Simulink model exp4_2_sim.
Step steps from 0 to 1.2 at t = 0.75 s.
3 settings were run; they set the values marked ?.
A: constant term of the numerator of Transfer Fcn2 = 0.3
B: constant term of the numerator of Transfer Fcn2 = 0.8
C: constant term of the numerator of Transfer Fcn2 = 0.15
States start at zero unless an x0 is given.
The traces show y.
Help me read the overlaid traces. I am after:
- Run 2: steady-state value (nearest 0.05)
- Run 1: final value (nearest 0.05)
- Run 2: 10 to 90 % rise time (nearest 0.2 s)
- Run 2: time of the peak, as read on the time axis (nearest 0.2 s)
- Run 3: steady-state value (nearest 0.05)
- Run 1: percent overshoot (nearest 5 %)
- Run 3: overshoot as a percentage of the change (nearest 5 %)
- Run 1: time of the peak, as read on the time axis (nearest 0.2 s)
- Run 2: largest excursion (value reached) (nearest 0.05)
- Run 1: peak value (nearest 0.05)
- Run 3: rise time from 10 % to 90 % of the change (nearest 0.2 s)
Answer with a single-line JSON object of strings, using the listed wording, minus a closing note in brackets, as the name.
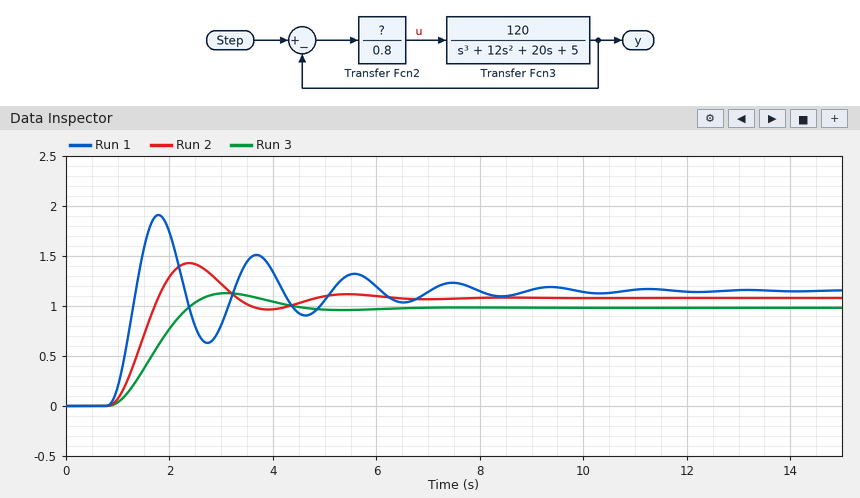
{"Run 2: steady-state value": "1.10", "Run 1: final value": "1.15", "Run 2: 10 to 90 % rise time": "0.6 s", "Run 2: time of the peak, as read on the time axis": "2.4 s", "Run 3: steady-state value": "1.00", "Run 1: percent overshoot": "65 %", "Run 3: overshoot as a percentage of the change": "15 %", "Run 1: time of the peak, as read on the time axis": "1.8 s", "Run 2: largest excursion (value reached)": "1.45", "Run 1: peak value": "1.90", "Run 3: rise time from 10 % to 90 % of the change": "1.0 s"}
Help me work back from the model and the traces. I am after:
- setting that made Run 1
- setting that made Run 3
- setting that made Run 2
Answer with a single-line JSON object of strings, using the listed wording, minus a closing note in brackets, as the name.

{"setting that made Run 1": "B", "setting that made Run 3": "C", "setting that made Run 2": "A"}
